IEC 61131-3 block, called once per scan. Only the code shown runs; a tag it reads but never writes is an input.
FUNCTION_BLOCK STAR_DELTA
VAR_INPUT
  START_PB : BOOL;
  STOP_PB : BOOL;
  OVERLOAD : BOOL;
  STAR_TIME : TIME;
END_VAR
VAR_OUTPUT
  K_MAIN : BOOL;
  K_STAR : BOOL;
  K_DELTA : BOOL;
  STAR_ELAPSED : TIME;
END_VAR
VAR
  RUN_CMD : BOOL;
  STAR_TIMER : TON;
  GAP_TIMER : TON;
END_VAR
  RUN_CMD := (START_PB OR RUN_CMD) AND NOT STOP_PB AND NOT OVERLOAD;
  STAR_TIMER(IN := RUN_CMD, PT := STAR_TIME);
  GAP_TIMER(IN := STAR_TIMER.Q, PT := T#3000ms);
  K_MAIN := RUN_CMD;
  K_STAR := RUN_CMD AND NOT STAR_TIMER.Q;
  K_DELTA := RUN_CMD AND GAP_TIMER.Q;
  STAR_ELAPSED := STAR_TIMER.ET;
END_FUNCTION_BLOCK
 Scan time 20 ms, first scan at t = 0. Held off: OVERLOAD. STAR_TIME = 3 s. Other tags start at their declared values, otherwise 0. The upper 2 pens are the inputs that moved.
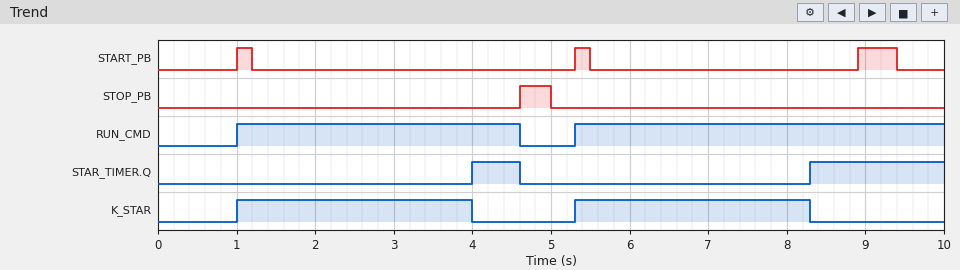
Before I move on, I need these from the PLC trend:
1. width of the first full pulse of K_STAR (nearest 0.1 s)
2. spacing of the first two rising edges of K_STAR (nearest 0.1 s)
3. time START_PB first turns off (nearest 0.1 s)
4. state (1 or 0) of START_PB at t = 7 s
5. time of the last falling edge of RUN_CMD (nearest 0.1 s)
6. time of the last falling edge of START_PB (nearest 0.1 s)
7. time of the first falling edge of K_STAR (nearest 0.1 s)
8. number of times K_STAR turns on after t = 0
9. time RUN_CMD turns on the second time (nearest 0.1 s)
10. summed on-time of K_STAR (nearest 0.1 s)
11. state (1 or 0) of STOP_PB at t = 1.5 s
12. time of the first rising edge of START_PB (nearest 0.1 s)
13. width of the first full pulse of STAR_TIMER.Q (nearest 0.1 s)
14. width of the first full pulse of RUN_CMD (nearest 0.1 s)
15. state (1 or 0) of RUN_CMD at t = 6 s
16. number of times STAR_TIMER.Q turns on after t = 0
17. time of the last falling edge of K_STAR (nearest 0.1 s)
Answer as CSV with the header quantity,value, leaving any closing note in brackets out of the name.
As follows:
quantity,value
width of the first full pulse of K_STAR,3.0 s
spacing of the first two rising edges of K_STAR,4.3 s
time START_PB first turns off,1.2 s
state (1 or 0) of START_PB at t = 7 s,0
time of the last falling edge of RUN_CMD,4.6 s
time of the last falling edge of START_PB,9.4 s
time of the first falling edge of K_STAR,4.0 s
number of times K_STAR turns on after t = 0,2
time RUN_CMD turns on the second time,5.3 s
summed on-time of K_STAR,6.0 s
state (1 or 0) of STOP_PB at t = 1.5 s,0
time of the first rising edge of START_PB,1.0 s
width of the first full pulse of STAR_TIMER.Q,0.6 s
width of the first full pulse of RUN_CMD,3.6 s
state (1 or 0) of RUN_CMD at t = 6 s,1
number of times STAR_TIMER.Q turns on after t = 0,2
time of the last falling edge of K_STAR,8.3 s
